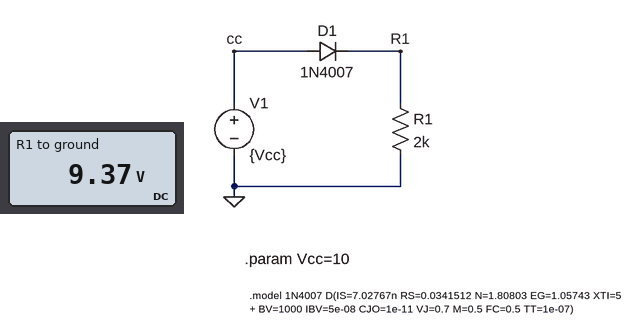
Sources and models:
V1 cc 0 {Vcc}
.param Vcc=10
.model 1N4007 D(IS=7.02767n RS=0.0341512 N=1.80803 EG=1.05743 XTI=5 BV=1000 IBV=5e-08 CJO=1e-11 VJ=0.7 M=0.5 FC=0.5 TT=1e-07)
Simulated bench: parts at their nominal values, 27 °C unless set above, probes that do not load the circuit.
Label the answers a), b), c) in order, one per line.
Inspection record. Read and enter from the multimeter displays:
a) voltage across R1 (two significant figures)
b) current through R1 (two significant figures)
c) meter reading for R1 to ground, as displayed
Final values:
a) 9.4 V
b) 4.7 mA
c) 9.37 V
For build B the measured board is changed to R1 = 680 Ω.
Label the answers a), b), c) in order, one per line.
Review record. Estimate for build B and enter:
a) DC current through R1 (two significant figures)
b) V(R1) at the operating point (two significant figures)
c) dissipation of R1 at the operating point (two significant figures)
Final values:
a) 14 mA
b) 9.3 V
c) 130 mW
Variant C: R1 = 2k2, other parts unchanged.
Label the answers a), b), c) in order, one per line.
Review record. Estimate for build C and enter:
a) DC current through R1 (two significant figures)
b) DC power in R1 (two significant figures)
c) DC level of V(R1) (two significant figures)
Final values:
a) 4.3 mA
b) 40 mW
c) 9.4 V
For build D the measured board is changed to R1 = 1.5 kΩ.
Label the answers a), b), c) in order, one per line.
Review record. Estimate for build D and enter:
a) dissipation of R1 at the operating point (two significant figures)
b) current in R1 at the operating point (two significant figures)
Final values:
a) 58 mW
b) 6.2 mA
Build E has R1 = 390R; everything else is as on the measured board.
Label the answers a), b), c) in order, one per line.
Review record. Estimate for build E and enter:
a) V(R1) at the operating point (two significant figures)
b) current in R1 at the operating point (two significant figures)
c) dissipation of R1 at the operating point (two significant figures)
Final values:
a) 9.3 V
b) 24 mA
c) 220 mW
